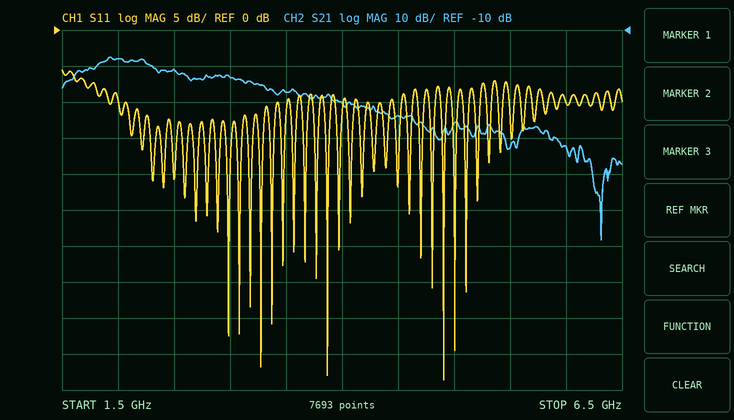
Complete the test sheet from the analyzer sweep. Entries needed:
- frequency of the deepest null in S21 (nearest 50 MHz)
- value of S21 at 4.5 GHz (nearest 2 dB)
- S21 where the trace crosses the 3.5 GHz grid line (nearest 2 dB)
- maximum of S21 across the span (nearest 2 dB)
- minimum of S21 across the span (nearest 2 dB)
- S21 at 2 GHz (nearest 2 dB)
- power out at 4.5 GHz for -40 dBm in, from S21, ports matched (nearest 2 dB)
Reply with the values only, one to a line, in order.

6.30 GHz
-34 dB
-28 dB
-18 dB
-68 dB
-18 dB
-74 dBm
